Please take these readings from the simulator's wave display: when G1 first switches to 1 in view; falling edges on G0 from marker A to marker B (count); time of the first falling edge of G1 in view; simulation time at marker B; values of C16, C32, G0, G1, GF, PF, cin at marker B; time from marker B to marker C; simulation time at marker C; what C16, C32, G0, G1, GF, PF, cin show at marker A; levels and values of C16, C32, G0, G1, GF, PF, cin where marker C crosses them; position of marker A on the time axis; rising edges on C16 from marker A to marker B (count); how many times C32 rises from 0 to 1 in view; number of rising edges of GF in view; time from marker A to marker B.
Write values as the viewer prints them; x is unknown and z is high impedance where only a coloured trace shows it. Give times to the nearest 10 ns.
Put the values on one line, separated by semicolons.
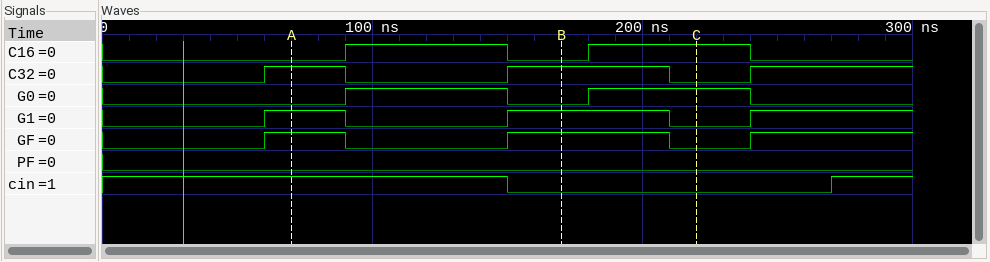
60 ns; 1; 90 ns; 170 ns; C16=0, C32=1, G0=0, G1=1, GF=1, PF=0, cin=0; 50 ns; 220 ns; C16=0, C32=1, G0=0, G1=1, GF=1, PF=0, cin=1; C16=1, C32=0, G0=1, G1=0, GF=0, PF=0, cin=0; 70 ns; 1; 3; 3; 100 ns
